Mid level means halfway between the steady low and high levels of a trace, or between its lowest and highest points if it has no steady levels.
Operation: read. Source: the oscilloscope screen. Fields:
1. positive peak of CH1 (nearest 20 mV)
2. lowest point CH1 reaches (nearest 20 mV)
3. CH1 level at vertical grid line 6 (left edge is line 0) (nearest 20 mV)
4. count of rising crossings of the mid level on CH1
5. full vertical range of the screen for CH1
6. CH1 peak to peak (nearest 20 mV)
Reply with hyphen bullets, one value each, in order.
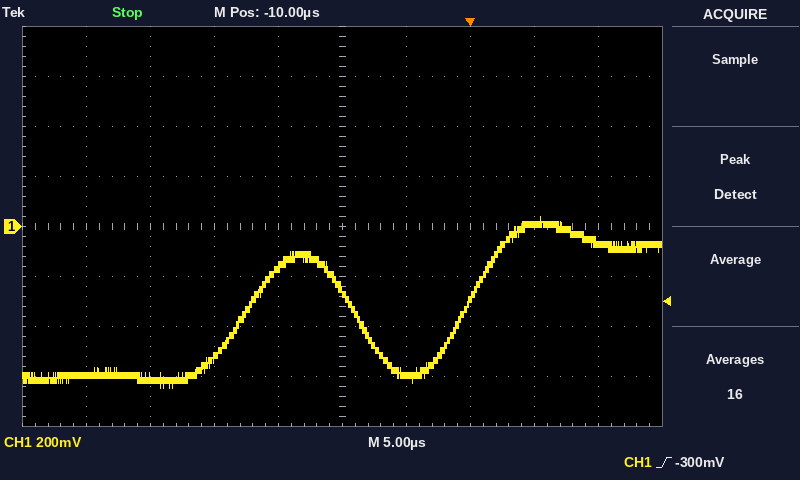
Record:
- 40 mV
- -640 mV
- -600 mV
- 2
- 1.6 V
- 680 mV
